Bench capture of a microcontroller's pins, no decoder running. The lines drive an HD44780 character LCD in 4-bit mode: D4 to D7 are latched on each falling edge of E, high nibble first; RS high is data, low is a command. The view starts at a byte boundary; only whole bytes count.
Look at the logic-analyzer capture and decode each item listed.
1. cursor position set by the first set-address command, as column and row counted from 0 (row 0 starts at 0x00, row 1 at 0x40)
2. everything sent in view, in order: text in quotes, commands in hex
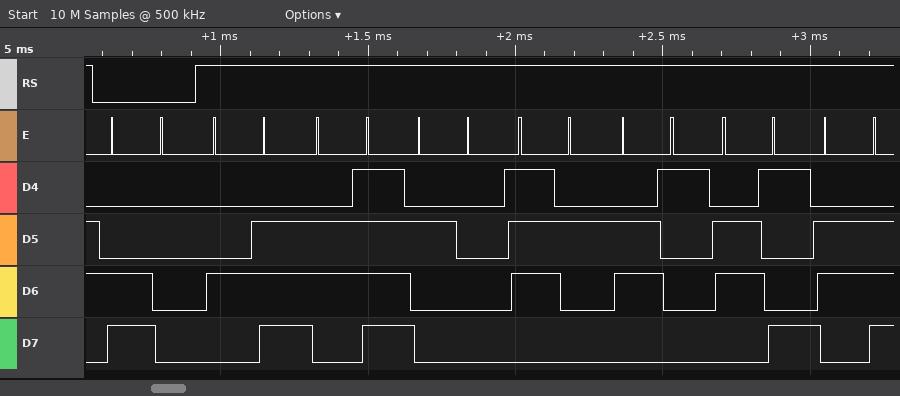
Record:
column 0, row 1
0xC0 "No rain"
